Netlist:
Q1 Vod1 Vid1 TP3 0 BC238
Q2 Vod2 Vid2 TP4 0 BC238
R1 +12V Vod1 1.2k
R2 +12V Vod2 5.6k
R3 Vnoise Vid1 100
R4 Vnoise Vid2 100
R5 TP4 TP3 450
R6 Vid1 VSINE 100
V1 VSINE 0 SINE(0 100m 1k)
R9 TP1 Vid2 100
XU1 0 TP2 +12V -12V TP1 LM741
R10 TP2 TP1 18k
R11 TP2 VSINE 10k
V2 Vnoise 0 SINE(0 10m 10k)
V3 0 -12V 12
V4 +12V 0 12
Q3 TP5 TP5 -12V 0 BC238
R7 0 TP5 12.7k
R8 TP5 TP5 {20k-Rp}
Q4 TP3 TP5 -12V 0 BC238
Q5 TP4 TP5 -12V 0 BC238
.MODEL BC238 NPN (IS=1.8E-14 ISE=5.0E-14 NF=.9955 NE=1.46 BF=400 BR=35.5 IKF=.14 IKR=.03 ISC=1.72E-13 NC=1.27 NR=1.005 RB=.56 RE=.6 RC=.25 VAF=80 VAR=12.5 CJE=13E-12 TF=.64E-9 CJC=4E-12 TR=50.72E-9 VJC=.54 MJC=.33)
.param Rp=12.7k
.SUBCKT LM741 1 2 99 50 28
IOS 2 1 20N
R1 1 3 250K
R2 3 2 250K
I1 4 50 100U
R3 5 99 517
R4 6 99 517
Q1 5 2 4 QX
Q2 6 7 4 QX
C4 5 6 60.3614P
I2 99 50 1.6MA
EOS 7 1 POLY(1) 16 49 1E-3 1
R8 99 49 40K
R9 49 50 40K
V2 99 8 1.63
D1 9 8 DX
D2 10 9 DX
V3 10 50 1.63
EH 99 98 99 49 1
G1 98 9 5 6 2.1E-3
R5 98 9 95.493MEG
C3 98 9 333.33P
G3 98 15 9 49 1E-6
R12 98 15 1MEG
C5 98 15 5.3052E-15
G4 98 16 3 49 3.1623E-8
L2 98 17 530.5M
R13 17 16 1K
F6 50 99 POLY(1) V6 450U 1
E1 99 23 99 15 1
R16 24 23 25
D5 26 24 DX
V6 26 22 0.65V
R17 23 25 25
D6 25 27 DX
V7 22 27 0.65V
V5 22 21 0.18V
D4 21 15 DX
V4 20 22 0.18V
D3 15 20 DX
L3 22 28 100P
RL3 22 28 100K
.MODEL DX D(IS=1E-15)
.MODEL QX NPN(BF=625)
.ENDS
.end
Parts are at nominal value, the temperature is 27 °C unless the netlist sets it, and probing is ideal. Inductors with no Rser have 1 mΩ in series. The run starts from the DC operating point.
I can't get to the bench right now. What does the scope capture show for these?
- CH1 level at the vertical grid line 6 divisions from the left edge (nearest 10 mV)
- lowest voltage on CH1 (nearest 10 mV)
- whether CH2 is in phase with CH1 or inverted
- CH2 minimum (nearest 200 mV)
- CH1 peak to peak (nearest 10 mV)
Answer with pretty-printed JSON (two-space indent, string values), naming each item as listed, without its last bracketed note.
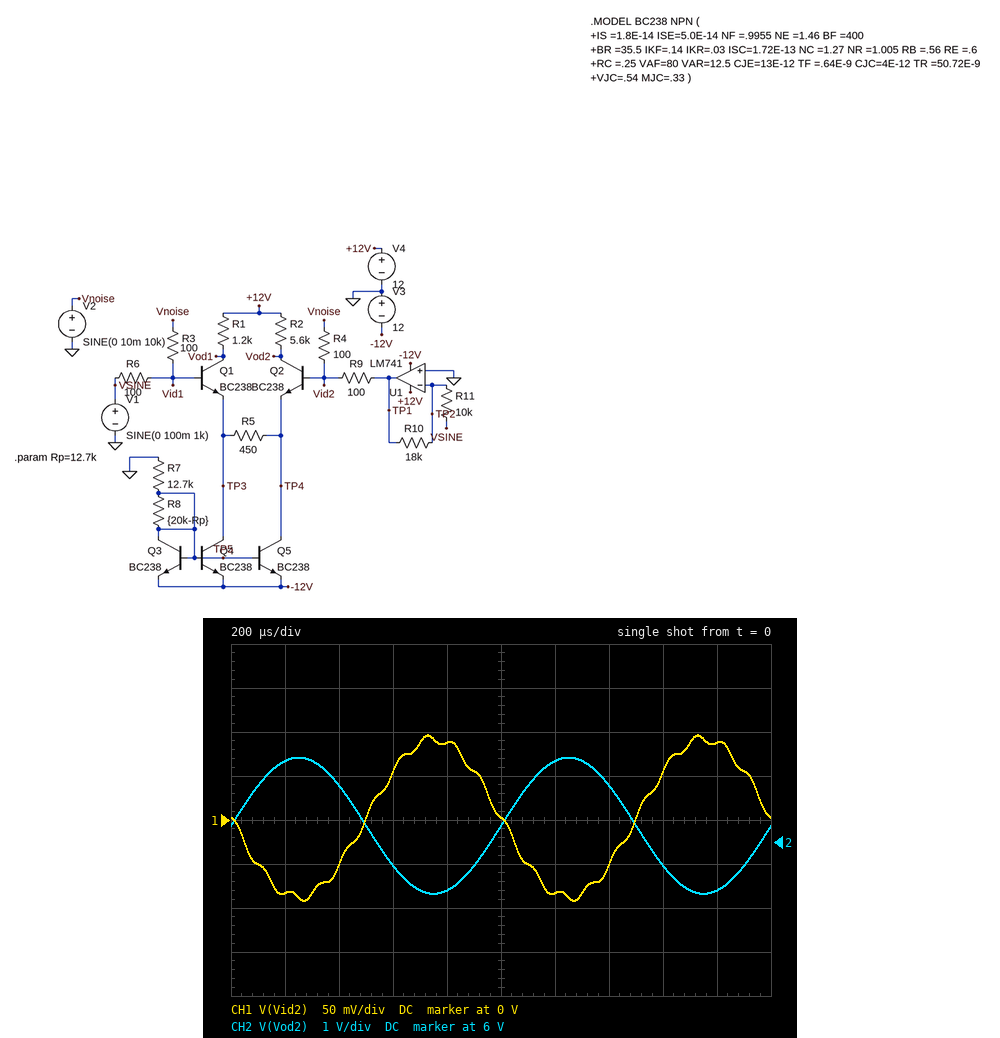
{
  "CH1 level at the vertical grid line 6 divisions from the left edge": "-80 mV",
  "lowest voltage on CH1": "-90 mV",
  "whether CH2 is in phase with CH1 or inverted": "inverted",
  "CH2 minimum": "4.8 V",
  "CH1 peak to peak": "190 mV"
}
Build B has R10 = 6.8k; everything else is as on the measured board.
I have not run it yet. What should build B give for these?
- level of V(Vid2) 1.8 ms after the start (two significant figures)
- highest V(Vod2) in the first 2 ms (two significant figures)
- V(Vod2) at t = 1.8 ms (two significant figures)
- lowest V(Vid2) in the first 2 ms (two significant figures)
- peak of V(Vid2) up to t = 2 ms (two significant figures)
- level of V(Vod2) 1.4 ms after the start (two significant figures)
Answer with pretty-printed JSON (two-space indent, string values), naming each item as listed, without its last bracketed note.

{
  "level of V(Vid2) 1.8 ms after the start": "33 mV",
  "highest V(Vod2) in the first 2 ms": "7.3 V",
  "V(Vod2) at t = 1.8 ms": "5.5 V",
  "lowest V(Vid2) in the first 2 ms": "-38 mV",
  "peak of V(Vid2) up to t = 2 ms": "40 mV",
  "level of V(Vod2) 1.4 ms after the start": "6.9 V"
}
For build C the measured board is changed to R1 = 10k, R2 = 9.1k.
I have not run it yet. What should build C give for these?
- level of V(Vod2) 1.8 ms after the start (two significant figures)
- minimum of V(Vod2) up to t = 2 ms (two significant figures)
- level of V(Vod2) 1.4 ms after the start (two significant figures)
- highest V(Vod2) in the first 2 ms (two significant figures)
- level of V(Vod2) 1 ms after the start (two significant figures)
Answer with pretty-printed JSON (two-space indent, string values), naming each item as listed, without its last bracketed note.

{
  "level of V(Vod2) 1.8 ms after the start": "450 mV",
  "minimum of V(Vod2) up to t = 2 ms": "330 mV",
  "level of V(Vod2) 1.4 ms after the start": "4.3 V",
  "highest V(Vod2) in the first 2 ms": "5.3 V",
  "level of V(Vod2) 1 ms after the start": "2.8 V"
}
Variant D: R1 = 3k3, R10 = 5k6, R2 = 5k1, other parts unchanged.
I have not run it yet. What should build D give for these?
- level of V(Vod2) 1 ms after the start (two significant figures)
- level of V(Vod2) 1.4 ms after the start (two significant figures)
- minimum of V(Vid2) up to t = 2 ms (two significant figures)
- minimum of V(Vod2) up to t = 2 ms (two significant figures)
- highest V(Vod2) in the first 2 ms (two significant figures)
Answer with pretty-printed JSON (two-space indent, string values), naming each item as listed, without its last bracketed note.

{
  "level of V(Vod2) 1 ms after the start": "6.9 V",
  "level of V(Vod2) 1.4 ms after the start": "7.3 V",
  "minimum of V(Vid2) up to t = 2 ms": "-32 mV",
  "minimum of V(Vod2) up to t = 2 ms": "6.1 V",
  "highest V(Vod2) in the first 2 ms": "7.7 V"
}
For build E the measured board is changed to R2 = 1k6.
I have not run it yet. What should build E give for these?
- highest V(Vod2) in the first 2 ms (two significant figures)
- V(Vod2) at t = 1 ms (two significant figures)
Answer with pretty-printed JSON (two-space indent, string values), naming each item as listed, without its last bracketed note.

{
  "highest V(Vod2) in the first 2 ms": "11 V",
  "V(Vod2) at t = 1 ms": "10 V"
}
